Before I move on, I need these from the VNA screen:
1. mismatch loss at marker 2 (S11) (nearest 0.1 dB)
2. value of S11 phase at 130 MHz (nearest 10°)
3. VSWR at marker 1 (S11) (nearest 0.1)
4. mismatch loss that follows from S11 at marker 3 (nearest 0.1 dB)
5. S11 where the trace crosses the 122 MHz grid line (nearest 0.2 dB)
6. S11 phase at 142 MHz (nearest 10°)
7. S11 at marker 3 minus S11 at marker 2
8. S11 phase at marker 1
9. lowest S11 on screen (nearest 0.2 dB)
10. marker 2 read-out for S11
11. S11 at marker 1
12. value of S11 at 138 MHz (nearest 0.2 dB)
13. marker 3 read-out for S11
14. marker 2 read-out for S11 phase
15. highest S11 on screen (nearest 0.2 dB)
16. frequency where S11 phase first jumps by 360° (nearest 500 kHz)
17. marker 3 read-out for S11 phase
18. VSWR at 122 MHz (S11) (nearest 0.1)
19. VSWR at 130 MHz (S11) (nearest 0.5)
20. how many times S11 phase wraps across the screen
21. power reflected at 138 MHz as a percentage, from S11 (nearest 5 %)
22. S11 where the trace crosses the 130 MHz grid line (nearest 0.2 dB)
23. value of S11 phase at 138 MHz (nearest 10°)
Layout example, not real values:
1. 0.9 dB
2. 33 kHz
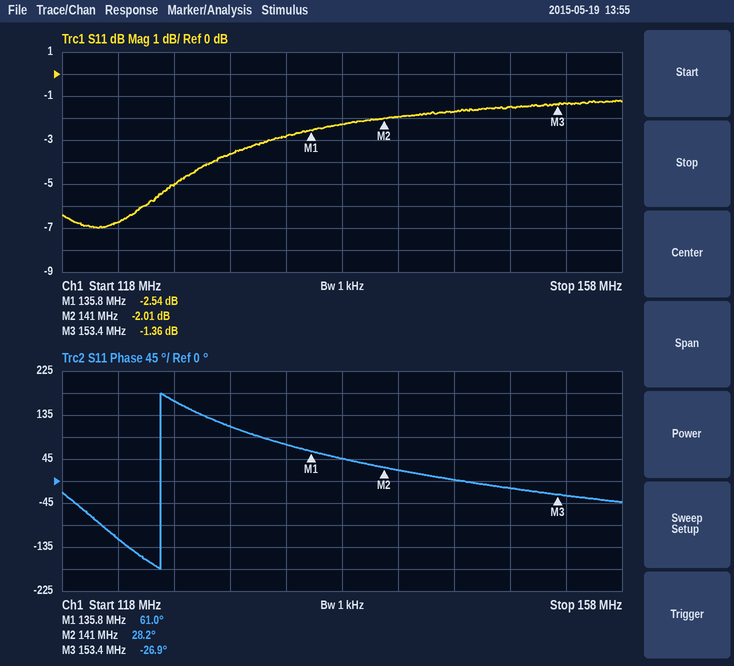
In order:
1. 4.3 dB
2. 110°
3. 6.9
4. 5.7 dB
5. -6.8 dB
6. 20°
7. 0.65 dB
8. 61.0°
9. -7.0 dB
10. -2.01 dB
11. -2.54 dB
12. -2.2 dB
13. -1.36 dB
14. 28.2°
15. -1.2 dB
16. 125.0 MHz
17. -26.9°
18. 2.7
19. 5.0
20. 1
21. 60 %
22. -3.6 dB
23. 50°
